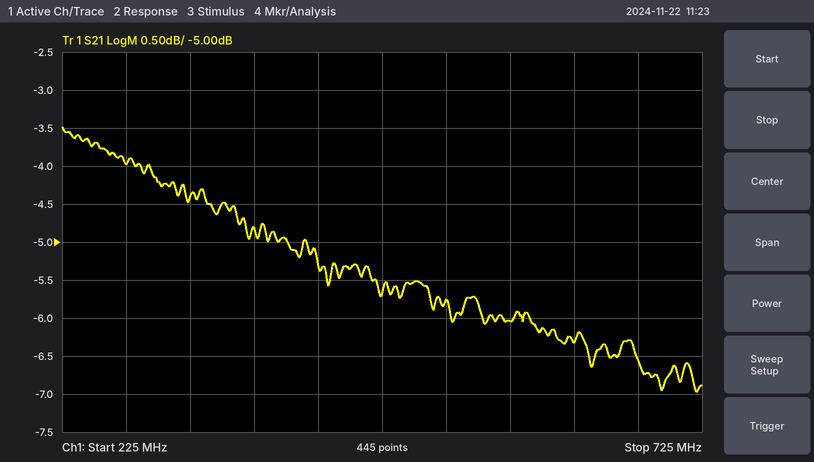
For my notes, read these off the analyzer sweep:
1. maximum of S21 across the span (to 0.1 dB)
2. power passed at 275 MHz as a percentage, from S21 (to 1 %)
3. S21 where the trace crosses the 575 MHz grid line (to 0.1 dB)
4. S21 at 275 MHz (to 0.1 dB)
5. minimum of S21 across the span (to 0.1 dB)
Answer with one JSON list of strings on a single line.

["-3.5 dB", "40 %", "-6.0 dB", "-4.0 dB", "-7.0 dB"]
